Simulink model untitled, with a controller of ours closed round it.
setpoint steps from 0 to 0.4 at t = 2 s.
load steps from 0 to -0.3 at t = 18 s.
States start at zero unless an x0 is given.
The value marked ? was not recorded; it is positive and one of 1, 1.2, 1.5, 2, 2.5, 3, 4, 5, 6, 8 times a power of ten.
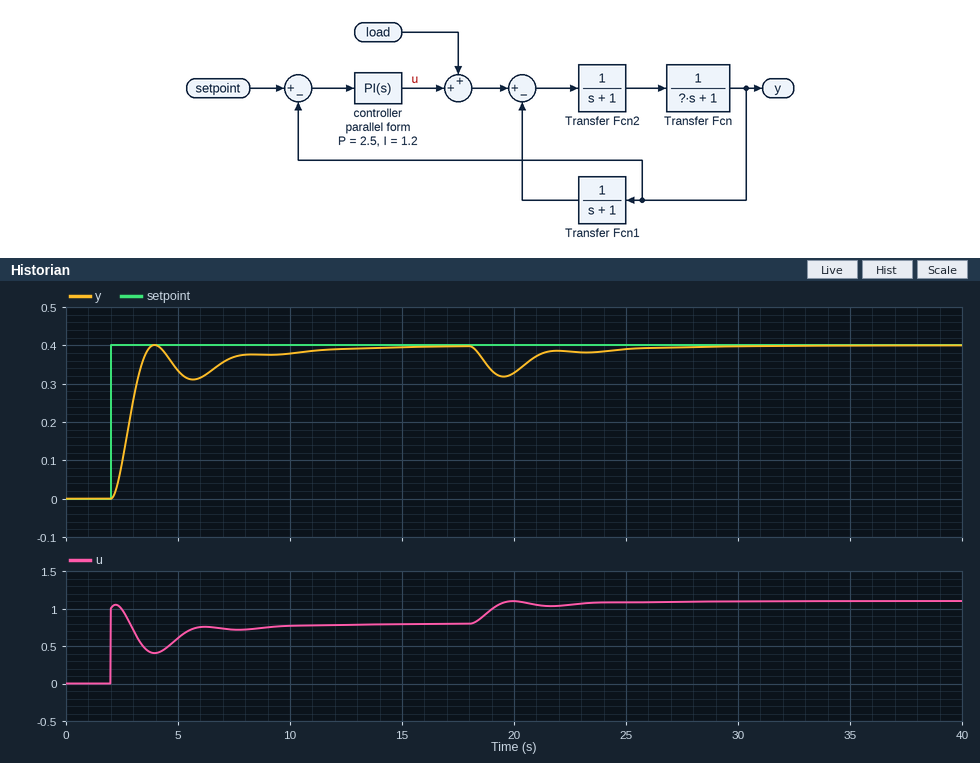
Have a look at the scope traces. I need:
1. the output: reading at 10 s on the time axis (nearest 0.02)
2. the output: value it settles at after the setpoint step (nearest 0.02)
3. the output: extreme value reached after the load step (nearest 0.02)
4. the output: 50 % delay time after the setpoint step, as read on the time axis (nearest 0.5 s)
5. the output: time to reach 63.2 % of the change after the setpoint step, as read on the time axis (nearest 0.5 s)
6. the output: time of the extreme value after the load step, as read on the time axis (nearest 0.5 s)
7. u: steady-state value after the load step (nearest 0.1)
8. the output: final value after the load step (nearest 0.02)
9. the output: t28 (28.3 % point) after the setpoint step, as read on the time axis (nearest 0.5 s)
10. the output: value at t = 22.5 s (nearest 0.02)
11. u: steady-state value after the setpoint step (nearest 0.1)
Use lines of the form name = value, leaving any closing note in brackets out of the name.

the output: reading at 10 s on the time axis = 0.38
the output: value it settles at after the setpoint step = 0.40
the output: extreme value reached after the load step = 0.32
the output: 50 % delay time after the setpoint step, as read on the time axis = 3.0 s
the output: time to reach 63.2 % of the change after the setpoint step, as read on the time axis = 3.0 s
the output: time of the extreme value after the load step, as read on the time axis = 19.5 s
u: steady-state value after the load step = 1.1
the output: final value after the load step = 0.40
the output: t28 (28.3 % point) after the setpoint step, as read on the time axis = 2.5 s
the output: value at t = 22.5 s = 0.38
u: steady-state value after the setpoint step = 0.8
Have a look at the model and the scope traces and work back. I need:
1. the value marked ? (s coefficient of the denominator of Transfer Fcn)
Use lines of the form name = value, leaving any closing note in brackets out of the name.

the value marked ? = 1
